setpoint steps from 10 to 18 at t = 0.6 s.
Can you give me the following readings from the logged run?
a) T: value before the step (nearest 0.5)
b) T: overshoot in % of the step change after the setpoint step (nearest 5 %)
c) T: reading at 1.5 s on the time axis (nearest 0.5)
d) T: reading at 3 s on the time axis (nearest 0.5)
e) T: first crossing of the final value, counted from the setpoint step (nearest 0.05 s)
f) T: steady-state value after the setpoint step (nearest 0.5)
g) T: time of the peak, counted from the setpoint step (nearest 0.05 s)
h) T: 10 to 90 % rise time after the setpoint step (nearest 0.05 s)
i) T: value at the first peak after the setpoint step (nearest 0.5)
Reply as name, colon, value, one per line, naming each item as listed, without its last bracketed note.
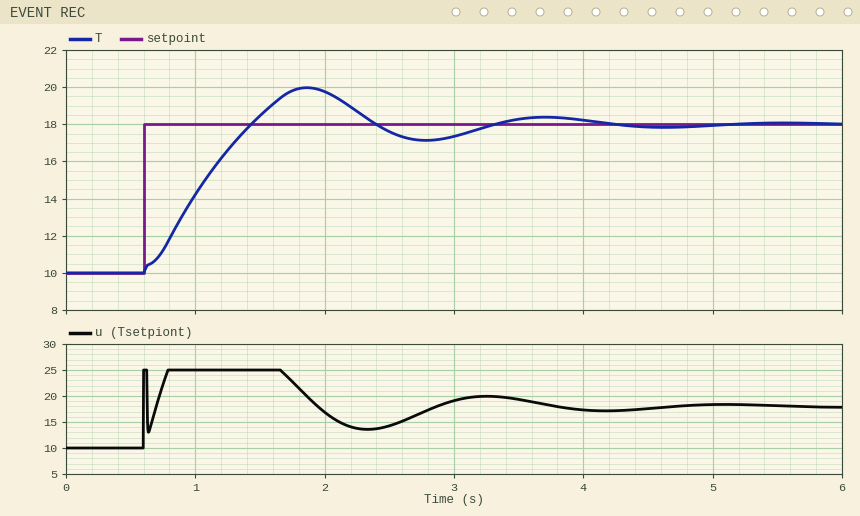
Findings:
T: value before the step: 10.0
T: overshoot in % of the step change after the setpoint step: 25 %
T: reading at 1.5 s on the time axis: 18.5
T: reading at 3 s on the time axis: 17.5
T: first crossing of the final value, counted from the setpoint step: 0.85 s
T: steady-state value after the setpoint step: 18.0
T: time of the peak, counted from the setpoint step: 1.25 s
T: 10 to 90 % rise time after the setpoint step: 0.60 s
T: value at the first peak after the setpoint step: 20.0
